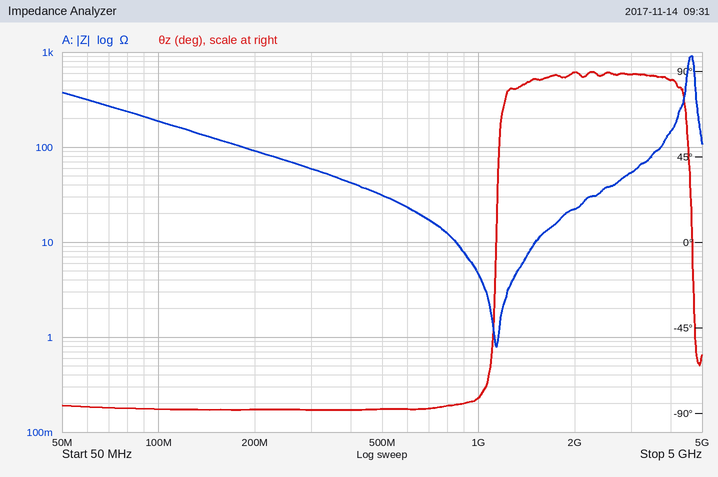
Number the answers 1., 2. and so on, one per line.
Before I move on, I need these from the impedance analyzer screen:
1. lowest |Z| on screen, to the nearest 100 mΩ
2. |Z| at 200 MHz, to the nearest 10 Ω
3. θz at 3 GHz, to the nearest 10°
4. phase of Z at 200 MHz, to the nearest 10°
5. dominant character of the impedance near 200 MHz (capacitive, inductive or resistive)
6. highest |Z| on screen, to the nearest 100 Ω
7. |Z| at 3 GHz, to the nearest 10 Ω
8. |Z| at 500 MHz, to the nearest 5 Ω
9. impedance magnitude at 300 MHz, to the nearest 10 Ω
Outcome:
1. 800 mΩ
2. 90 Ω
3. 90°
4. -90°
5. capacitive
6. 900 Ω
7. 50 Ω
8. 30 Ω
9. 60 Ω
